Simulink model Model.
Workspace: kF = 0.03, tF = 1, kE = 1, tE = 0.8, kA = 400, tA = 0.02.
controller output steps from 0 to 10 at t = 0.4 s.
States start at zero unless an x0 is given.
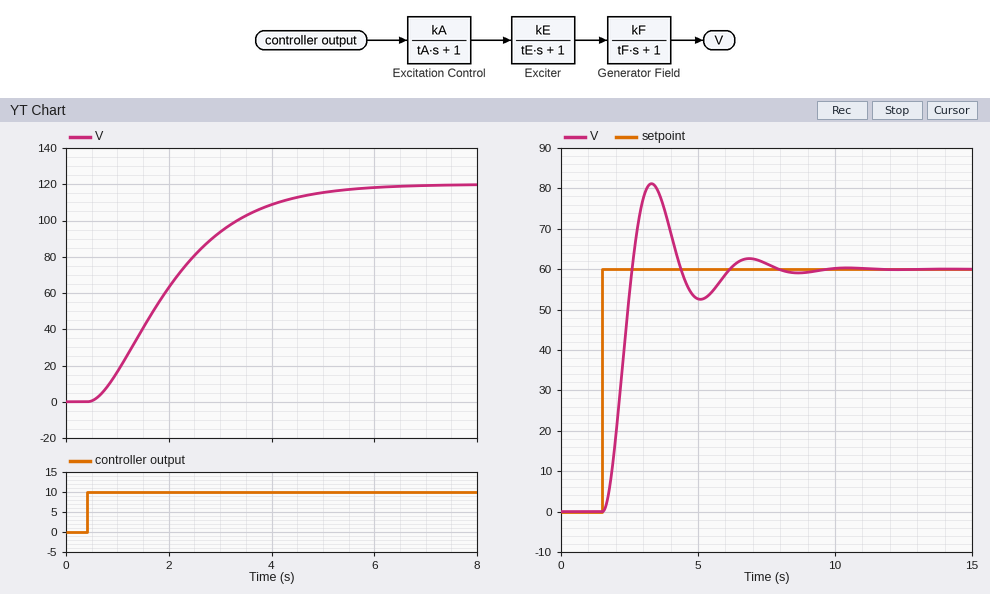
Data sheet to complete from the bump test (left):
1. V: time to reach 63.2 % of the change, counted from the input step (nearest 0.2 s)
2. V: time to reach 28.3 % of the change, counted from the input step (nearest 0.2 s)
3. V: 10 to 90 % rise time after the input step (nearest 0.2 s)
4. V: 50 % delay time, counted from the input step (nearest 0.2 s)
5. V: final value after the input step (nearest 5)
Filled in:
2.0 s
1.0 s
3.0 s
1.6 s
120
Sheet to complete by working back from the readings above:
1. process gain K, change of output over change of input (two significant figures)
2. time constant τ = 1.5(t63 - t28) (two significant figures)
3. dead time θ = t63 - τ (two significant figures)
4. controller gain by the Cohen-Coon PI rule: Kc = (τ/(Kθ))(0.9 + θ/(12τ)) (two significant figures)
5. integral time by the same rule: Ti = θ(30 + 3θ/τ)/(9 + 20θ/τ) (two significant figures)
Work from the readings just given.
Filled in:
12
1.5 s
0.50 s
0.23
0.99 s
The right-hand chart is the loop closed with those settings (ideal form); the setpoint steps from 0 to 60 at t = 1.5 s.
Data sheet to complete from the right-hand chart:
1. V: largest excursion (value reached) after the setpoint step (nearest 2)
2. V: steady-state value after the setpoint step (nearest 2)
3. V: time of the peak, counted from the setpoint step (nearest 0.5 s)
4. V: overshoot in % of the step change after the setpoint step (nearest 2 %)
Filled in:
82
60
2.0 s
36 %
